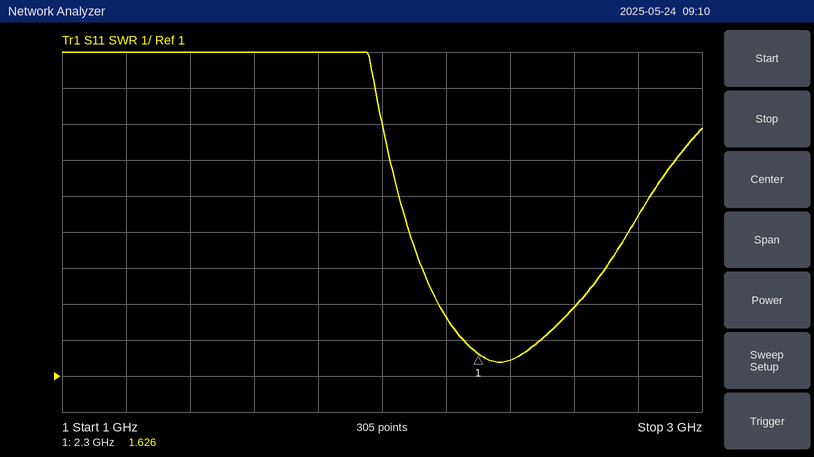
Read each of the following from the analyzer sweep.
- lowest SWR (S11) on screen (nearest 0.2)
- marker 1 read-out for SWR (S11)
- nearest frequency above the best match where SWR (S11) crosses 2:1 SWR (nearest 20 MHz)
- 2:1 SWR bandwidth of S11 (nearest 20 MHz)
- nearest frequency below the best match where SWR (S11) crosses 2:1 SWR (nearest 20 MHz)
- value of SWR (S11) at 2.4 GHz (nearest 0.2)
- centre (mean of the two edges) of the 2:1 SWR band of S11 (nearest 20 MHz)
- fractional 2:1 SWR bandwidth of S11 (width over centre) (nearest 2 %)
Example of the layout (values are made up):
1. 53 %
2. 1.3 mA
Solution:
1. 1.4
2. 1.626
3. 2.50 GHz
4. 240 MHz
5. 2.26 GHz
6. 1.4
7. 2.38 GHz
8. 10 %
